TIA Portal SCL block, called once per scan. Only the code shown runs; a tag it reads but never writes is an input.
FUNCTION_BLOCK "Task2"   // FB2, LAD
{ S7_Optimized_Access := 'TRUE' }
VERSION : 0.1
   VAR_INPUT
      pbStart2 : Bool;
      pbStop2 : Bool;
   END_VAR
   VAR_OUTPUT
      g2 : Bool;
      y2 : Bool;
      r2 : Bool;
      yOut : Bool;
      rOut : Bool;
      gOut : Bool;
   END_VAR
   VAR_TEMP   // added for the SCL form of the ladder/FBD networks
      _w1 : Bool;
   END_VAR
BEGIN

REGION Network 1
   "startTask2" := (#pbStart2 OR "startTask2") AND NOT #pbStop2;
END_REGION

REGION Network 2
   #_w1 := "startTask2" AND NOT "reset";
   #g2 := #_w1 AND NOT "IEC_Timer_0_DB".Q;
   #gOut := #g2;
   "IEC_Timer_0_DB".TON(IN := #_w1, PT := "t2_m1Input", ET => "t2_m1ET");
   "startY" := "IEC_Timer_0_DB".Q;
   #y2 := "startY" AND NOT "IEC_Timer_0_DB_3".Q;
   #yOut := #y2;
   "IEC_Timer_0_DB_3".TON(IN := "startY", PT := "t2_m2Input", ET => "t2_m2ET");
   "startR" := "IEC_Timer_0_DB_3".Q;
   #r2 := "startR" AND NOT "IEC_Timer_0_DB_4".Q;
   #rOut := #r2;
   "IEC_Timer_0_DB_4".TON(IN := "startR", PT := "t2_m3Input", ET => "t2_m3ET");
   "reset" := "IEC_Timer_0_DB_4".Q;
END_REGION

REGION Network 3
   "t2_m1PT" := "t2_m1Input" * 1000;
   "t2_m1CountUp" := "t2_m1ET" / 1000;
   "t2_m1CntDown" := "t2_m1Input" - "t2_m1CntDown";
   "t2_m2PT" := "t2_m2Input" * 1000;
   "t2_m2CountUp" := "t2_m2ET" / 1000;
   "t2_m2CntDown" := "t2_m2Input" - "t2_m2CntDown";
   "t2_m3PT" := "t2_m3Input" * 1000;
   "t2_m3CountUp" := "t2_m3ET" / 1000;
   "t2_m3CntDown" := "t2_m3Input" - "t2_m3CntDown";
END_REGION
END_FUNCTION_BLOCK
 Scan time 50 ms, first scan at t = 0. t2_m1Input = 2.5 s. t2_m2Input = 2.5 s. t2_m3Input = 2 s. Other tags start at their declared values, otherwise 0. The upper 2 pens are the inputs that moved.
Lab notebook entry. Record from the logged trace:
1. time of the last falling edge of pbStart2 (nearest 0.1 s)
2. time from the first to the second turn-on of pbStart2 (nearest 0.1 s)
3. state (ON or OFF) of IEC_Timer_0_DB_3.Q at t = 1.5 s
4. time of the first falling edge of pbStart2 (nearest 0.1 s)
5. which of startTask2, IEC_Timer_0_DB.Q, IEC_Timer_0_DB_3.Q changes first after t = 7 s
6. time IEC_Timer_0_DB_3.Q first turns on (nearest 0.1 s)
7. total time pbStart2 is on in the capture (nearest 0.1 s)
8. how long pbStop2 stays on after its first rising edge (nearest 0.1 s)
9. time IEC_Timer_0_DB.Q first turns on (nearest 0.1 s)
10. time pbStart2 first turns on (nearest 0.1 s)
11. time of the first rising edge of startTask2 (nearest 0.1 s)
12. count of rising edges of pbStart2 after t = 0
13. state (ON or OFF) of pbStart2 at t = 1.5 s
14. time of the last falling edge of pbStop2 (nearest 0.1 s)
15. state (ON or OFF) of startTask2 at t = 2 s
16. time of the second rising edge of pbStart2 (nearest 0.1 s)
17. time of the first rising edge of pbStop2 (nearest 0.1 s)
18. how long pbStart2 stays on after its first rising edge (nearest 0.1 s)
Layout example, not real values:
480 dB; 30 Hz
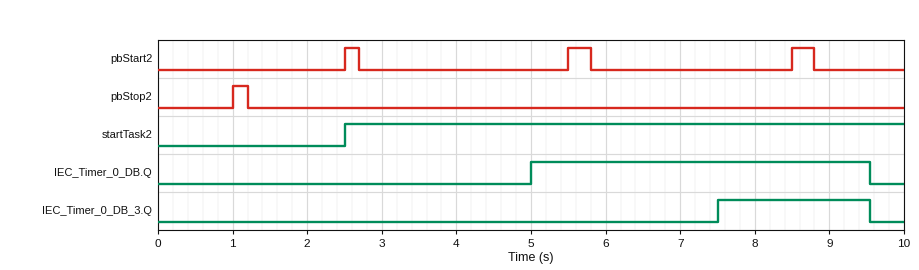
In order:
8.8 s; 3.0 s; OFF; 2.7 s; IEC_Timer_0_DB_3.Q; 7.5 s; 0.8 s; 0.2 s; 5.0 s; 2.5 s; 2.5 s; 3; OFF; 1.2 s; OFF; 5.5 s; 1.0 s; 0.2 s
